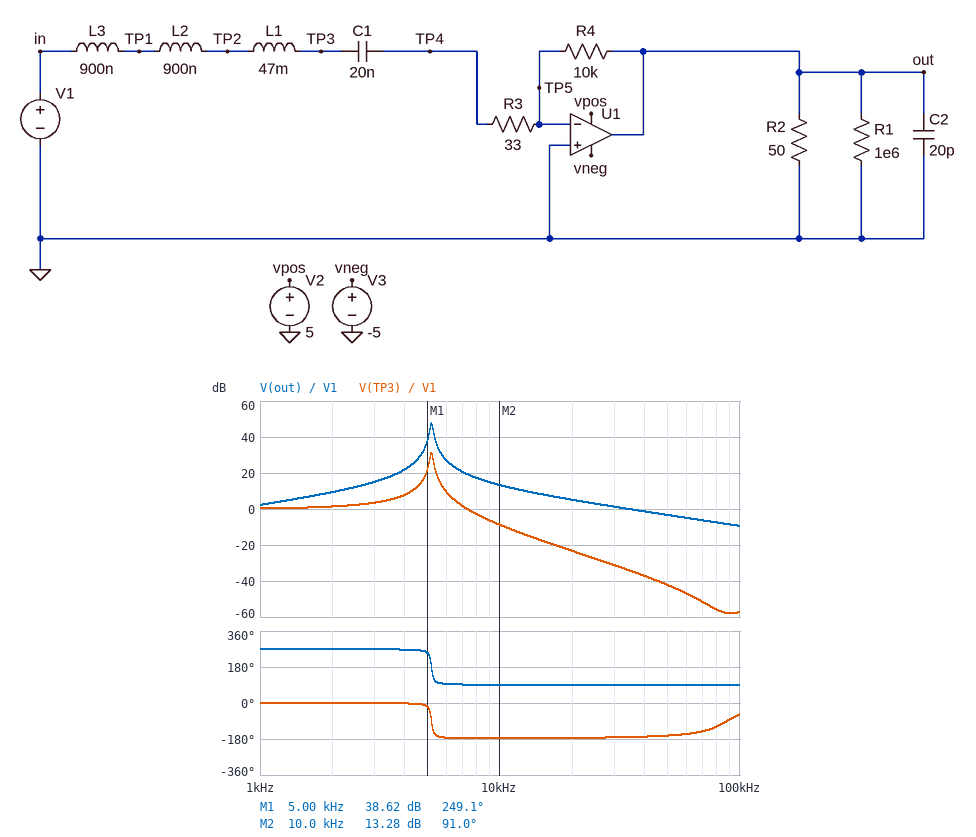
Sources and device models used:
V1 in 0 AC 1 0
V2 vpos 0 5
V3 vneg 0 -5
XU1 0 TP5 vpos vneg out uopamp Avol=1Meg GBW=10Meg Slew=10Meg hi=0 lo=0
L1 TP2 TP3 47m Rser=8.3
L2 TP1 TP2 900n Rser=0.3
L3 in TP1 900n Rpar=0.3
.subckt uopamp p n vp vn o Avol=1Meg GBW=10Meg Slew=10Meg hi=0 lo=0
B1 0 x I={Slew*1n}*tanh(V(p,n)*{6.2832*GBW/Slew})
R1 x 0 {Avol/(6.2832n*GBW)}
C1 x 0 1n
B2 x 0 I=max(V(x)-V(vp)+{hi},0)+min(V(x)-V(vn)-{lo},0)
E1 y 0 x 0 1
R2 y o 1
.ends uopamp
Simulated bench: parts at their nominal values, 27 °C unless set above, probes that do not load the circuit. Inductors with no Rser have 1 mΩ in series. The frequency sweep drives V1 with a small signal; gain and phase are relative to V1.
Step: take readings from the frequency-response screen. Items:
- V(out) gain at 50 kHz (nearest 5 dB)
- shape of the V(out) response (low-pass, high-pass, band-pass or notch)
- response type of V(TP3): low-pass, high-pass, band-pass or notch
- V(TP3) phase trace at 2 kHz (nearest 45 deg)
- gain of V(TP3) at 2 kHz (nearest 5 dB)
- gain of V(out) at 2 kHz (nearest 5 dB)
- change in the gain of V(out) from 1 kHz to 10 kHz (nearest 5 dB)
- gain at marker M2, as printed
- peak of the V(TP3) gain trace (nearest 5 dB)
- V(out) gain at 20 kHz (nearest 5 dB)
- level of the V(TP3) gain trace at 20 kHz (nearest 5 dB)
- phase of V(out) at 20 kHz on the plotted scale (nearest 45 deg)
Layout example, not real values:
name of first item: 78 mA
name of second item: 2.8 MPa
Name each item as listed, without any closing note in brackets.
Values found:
V(out) gain at 50 kHz: -5 dB
shape of the V(out) response: band-pass
response type of V(TP3): low-pass, high-pass, band-pass or notch: low-pass
V(TP3) phase trace at 2 kHz: 0 deg
gain of V(TP3) at 2 kHz: 0 dB
gain of V(out) at 2 kHz: 10 dB
change in the gain of V(out) from 1 kHz to 10 kHz: 10 dB
gain at marker M2, as printed: 13.28 dB
peak of the V(TP3) gain trace: 30 dB
V(out) gain at 20 kHz: 5 dB
level of the V(TP3) gain trace at 20 kHz: -25 dB
phase of V(out) at 20 kHz on the plotted scale: 90 deg
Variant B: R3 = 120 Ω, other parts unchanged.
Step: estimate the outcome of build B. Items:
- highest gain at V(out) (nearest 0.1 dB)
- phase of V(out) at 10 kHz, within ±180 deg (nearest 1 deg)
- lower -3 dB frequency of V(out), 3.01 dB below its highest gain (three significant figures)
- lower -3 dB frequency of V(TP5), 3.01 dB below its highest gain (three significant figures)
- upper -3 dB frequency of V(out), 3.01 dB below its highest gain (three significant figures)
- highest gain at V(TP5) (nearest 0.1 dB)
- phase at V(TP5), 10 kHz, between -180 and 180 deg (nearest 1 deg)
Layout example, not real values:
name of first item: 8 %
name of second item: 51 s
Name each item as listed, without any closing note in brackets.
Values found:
highest gain at V(out): 37.8 dB
phase of V(out) at 10 kHz, within ±180 deg: 93 deg
lower -3 dB frequency of V(out), 3.01 dB below its highest gain: 4.97 kHz
lower -3 dB frequency of V(TP5), 3.01 dB below its highest gain: 4.99 kHz
upper -3 dB frequency of V(out), 3.01 dB below its highest gain: 5.40 kHz
highest gain at V(TP5): -27.7 dB
phase at V(TP5), 10 kHz, between -180 and 180 deg: 3 deg
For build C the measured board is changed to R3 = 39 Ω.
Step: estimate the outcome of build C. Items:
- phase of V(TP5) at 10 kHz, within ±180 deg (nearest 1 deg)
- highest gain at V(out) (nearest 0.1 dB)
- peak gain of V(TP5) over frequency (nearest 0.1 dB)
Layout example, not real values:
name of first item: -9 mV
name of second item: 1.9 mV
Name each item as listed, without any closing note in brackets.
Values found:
phase of V(TP5) at 10 kHz, within ±180 deg: 1 deg
highest gain at V(out): 46.4 dB
peak gain of V(TP5) over frequency: -19.1 dB
